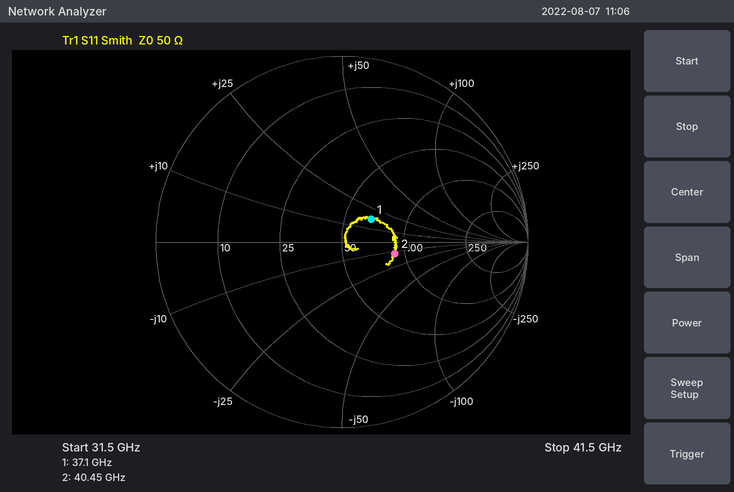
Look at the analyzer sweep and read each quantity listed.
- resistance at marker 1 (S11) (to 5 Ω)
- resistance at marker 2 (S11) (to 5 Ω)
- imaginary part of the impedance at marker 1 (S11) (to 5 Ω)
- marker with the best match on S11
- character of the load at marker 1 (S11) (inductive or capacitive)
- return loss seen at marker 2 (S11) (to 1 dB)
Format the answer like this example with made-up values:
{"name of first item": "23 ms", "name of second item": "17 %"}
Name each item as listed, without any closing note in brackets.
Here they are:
{"resistance at marker 1 (S11)": "65 Ω", "resistance at marker 2 (S11)": "90 Ω", "imaginary part of the impedance at marker 1 (S11)": "+15 Ω", "marker with the best match on S11": "marker 1", "character of the load at marker 1 (S11)": "inductive", "return loss seen at marker 2 (S11)": "11 dB"}
